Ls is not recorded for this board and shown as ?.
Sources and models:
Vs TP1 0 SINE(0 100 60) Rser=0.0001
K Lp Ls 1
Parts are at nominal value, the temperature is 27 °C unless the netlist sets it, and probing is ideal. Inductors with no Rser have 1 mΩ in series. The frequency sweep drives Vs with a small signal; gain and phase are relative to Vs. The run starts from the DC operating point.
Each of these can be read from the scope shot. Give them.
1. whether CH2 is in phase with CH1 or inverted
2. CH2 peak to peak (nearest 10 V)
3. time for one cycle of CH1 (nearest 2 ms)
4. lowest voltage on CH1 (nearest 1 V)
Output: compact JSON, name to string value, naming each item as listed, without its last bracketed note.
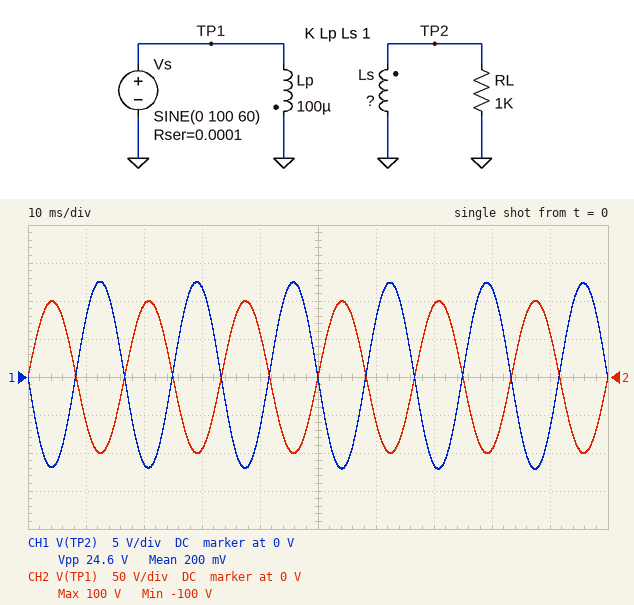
{"whether CH2 is in phase with CH1 or inverted": "inverted", "CH2 peak to peak": "200 V", "time for one cycle of CH1": "16 ms", "lowest voltage on CH1": "-12 V"}
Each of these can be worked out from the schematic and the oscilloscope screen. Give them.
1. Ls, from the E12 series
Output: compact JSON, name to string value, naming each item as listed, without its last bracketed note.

{"Ls, from the E12 series": "1.5 µH"}
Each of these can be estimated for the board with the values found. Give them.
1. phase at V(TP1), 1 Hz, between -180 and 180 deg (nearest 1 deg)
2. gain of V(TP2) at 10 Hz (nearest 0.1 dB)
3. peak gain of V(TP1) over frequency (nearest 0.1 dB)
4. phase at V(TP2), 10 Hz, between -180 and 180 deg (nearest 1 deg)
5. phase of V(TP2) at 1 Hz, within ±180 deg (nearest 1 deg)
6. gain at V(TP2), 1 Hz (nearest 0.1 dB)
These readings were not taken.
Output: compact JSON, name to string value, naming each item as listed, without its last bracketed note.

{"phase at V(TP1), 1 Hz, between -180 and 180 deg": "2 deg", "gain of V(TP2) at 10 Hz": "-18.4 dB", "peak gain of V(TP1) over frequency": "0 dB", "phase at V(TP2), 10 Hz, between -180 and 180 deg": "-170 deg", "phase of V(TP2) at 1 Hz, within ±180 deg": "-120 deg", "gain at V(TP2), 1 Hz": "-24.3 dB"}
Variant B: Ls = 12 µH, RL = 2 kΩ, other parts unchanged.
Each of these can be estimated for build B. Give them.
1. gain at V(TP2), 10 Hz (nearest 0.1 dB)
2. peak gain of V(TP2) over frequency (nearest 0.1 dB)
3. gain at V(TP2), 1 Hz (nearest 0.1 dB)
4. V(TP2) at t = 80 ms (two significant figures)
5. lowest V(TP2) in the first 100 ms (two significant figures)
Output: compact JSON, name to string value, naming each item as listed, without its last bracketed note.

{"gain at V(TP2), 10 Hz": "-9.3 dB", "peak gain of V(TP2) over frequency": "-9.2 dB", "gain at V(TP2), 1 Hz": "-15.3 dB", "V(TP2) at t = 80 ms": "33 V", "lowest V(TP2) in the first 100 ms": "-34 V"}
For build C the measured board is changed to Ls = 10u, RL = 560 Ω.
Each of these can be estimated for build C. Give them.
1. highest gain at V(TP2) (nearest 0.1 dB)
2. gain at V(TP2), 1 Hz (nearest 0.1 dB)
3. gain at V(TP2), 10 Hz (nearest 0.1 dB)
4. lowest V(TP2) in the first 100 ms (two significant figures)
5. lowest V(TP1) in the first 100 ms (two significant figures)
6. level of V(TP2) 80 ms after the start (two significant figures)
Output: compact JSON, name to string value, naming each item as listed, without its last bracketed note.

{"highest gain at V(TP2)": "-10.0 dB", "gain at V(TP2), 1 Hz": "-16.1 dB", "gain at V(TP2), 10 Hz": "-10.1 dB", "lowest V(TP2) in the first 100 ms": "-31 V", "lowest V(TP1) in the first 100 ms": "-100 V", "level of V(TP2) 80 ms after the start": "30 V"}
